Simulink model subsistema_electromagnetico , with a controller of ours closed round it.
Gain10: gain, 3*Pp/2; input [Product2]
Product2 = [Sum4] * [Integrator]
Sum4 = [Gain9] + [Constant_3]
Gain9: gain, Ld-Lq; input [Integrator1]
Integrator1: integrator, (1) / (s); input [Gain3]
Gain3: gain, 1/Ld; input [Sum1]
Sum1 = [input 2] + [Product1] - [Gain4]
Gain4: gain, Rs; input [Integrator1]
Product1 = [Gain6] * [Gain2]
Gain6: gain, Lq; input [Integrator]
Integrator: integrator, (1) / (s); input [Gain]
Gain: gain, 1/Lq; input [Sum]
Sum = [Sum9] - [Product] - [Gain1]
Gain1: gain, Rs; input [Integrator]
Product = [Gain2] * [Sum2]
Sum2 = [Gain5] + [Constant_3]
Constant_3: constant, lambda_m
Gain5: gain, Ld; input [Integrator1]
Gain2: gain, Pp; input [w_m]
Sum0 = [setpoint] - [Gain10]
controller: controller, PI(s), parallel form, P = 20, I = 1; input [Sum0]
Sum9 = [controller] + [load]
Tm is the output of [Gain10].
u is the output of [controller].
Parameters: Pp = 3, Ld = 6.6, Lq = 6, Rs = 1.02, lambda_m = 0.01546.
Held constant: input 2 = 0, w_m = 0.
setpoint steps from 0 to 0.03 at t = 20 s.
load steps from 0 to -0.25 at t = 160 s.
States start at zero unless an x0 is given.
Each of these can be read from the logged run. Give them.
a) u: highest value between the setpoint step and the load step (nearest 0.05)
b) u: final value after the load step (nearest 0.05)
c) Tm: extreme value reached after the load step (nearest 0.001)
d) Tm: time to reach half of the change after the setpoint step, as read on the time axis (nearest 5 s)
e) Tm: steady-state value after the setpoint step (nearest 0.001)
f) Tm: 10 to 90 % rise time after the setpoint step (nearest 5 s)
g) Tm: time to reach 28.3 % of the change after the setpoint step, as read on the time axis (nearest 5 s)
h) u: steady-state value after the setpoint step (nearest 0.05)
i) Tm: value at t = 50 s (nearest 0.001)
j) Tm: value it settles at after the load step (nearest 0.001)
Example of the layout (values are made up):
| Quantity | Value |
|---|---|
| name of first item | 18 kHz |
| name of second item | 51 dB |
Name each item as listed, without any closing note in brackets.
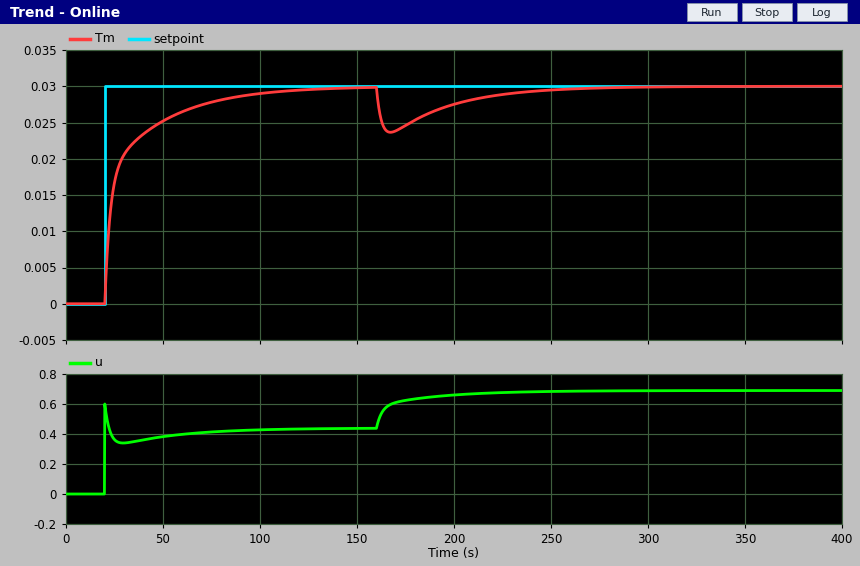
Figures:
| Quantity | Value |
|---|---|
| u: highest value between the setpoint step and the load step | 0.60 |
| u: final value after the load step | 0.70 |
| Tm: extreme value reached after the load step | 0.024 |
| Tm: time to reach half of the change after the setpoint step, as read on the time axis | 25 s |
| Tm: steady-state value after the setpoint step | 0.030 |
| Tm: 10 to 90 % rise time after the setpoint step | 45 s |
| Tm: time to reach 28.3 % of the change after the setpoint step, as read on the time axis | 20 s |
| u: steady-state value after the setpoint step | 0.45 |
| Tm: value at t = 50 s | 0.025 |
| Tm: value it settles at after the load step | 0.030 |
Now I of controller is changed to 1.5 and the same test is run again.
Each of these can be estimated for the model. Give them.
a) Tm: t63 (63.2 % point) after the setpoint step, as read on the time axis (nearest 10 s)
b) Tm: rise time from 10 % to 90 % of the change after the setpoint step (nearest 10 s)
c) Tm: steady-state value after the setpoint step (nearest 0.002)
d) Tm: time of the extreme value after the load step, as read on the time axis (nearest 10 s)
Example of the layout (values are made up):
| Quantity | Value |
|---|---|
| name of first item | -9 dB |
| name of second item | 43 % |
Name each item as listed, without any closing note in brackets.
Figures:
| Quantity | Value |
|---|---|
| Tm: t63 (63.2 % point) after the setpoint step, as read on the time axis | 30 s |
| Tm: rise time from 10 % to 90 % of the change after the setpoint step | 30 s |
| Tm: steady-state value after the setpoint step | 0.030 |
| Tm: time of the extreme value after the load step, as read on the time axis | 170 s |
